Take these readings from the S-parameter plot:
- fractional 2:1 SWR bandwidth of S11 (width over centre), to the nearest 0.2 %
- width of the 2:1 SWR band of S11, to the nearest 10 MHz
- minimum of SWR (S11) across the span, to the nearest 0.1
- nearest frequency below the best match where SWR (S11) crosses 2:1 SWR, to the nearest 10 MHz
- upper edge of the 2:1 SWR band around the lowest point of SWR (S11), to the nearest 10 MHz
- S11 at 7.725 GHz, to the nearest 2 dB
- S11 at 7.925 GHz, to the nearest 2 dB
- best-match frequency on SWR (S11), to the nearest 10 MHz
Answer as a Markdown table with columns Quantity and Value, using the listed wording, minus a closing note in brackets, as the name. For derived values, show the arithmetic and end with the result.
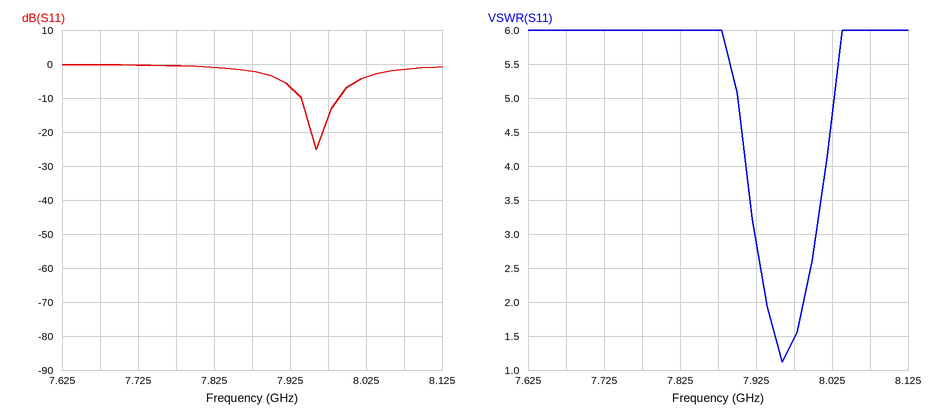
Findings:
| Quantity | Value |
|---|---|
| fractional 2:1 SWR bandwidth of S11 (width over centre), to the nearest 0.2 % | 50 MHz / 7.965 GHz ≈ 0.6 % |
| width of the 2:1 SWR band of S11, to the nearest 10 MHz | 7.99 GHz − 7.94 GHz = 50 MHz |
| minimum of SWR (S11) across the span, to the nearest 0.1 | 1.1 |
| nearest frequency below the best match where SWR (S11) crosses 2:1 SWR, to the nearest 10 MHz | 7.94 GHz |
| upper edge of the 2:1 SWR band around the lowest point of SWR (S11), to the nearest 10 MHz | 7.99 GHz |
| S11 at 7.725 GHz, to the nearest 2 dB | 0 dB |
| S11 at 7.925 GHz, to the nearest 2 dB | -6 dB |
| best-match frequency on SWR (S11), to the nearest 10 MHz | 7.96 GHz |
